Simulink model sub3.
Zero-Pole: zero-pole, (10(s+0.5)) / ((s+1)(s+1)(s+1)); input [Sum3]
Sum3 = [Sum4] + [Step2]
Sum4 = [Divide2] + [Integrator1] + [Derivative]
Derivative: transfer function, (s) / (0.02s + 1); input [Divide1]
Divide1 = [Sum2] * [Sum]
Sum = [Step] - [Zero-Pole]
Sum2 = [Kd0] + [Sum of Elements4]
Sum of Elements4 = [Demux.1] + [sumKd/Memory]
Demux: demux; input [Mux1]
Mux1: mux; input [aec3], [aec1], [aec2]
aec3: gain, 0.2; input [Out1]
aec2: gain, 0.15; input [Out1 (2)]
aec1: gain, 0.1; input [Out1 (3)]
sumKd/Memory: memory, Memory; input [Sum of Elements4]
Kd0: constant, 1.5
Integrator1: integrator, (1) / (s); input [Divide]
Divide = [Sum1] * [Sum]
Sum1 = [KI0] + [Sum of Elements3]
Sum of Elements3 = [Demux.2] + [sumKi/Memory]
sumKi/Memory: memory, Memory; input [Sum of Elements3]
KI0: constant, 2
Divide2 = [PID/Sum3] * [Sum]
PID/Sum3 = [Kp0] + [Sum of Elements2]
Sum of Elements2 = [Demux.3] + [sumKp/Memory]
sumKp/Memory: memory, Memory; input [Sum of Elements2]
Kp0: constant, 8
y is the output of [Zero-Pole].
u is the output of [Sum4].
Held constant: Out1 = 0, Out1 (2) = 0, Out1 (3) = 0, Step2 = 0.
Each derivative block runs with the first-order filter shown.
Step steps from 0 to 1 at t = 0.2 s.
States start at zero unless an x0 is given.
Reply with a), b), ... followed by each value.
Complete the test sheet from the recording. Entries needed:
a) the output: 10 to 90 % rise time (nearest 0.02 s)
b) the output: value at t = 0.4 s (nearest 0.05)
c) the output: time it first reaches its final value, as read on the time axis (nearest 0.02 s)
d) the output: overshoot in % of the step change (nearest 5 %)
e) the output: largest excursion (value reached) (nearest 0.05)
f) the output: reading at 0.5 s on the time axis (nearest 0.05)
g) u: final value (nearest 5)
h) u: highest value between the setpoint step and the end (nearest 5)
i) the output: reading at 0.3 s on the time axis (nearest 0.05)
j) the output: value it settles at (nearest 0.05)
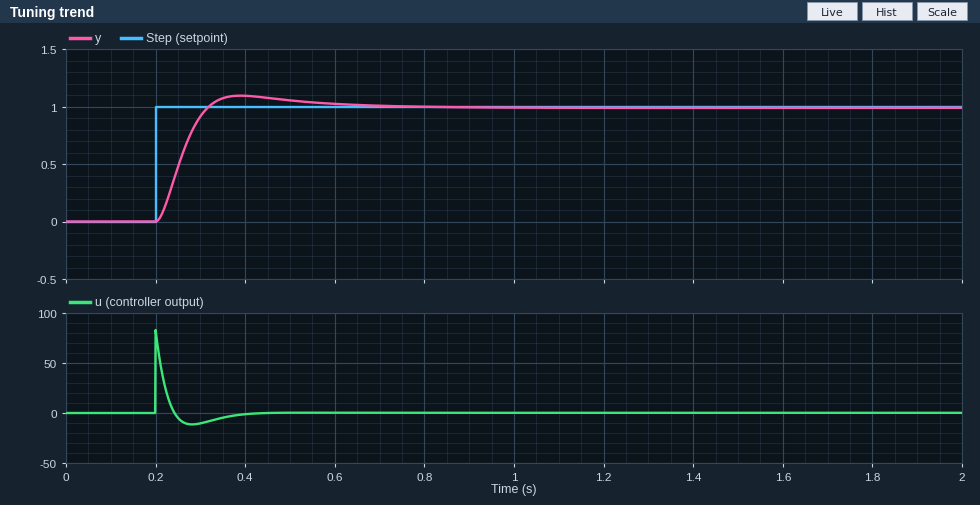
a) 0.08 s
b) 1.10
c) 0.32 s
d) 10 %
e) 1.10
f) 1.05
g) 0
h) 85
i) 0.90
j) 1.00
